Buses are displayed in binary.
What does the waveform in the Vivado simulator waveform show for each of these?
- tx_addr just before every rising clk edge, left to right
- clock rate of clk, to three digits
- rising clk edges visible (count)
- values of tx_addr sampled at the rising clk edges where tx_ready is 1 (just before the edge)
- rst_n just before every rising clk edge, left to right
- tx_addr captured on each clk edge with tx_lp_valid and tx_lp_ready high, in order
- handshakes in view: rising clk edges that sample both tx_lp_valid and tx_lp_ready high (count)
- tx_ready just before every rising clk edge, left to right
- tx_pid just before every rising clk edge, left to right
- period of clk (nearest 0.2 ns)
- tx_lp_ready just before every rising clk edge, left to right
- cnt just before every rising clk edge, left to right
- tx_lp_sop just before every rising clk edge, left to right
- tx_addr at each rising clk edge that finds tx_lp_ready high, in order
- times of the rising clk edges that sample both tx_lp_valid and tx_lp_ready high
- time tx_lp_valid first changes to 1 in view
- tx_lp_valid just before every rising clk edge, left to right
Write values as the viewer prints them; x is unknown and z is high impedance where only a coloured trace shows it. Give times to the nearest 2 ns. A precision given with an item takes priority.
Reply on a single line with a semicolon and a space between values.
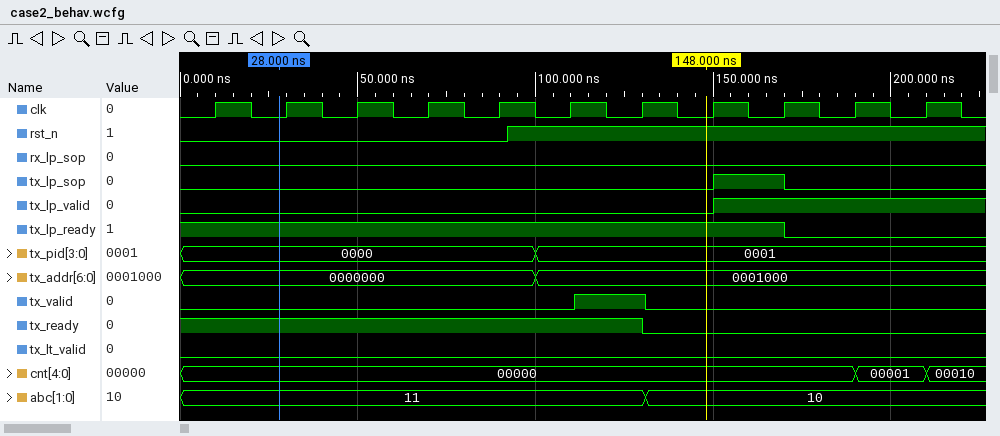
0000000, 0000000, 0000000, 0000000, 0000000, 0001000, 0001000, 0001000, 0001000, 0001000, 0001000; 50.0 MHz; 11; 0000000, 0000000, 0000000, 0000000, 0000000, 0001000, 0001000; 0 0 0 0 0 1 1 1 1 1 1; 0001000; 1; 1 1 1 1 1 1 1 0 0 0 0; 0000, 0000, 0000, 0000, 0000, 0001, 0001, 0001, 0001, 0001, 0001; 20 ns; 1 1 1 1 1 1 1 1 1 0 0; 00000, 00000, 00000, 00000, 00000, 00000, 00000, 00000, 00000, 00000, 00001; 0 0 0 0 0 0 0 0 1 0 0; 0000000, 0000000, 0000000, 0000000, 0000000, 0001000, 0001000, 0001000, 0001000; 170 ns; 150 ns; 0 0 0 0 0 0 0 0 1 1 1
